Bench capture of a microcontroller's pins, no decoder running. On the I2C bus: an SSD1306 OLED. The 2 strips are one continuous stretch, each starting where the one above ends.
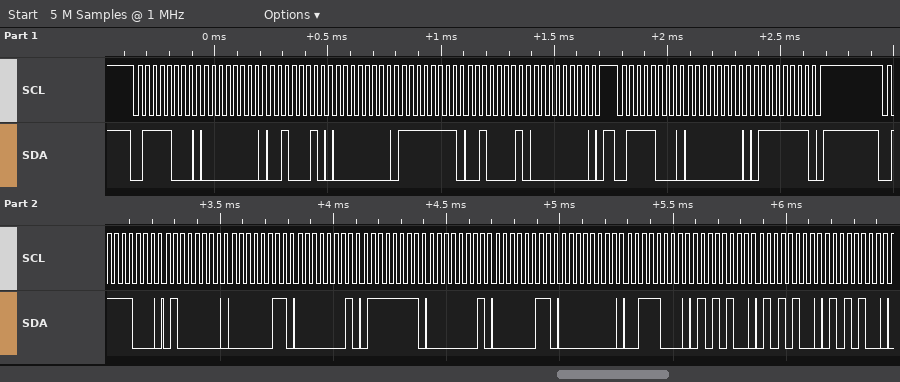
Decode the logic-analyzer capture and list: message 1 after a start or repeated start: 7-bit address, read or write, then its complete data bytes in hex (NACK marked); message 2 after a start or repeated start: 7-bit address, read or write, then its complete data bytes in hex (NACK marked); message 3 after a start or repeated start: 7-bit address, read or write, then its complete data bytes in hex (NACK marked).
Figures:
0x3C write: 00 22 00 FF 21 00
0x3C write: 00 7F
0x3C write: 40 03 01 7F 01 03 00 38 54 54 54
